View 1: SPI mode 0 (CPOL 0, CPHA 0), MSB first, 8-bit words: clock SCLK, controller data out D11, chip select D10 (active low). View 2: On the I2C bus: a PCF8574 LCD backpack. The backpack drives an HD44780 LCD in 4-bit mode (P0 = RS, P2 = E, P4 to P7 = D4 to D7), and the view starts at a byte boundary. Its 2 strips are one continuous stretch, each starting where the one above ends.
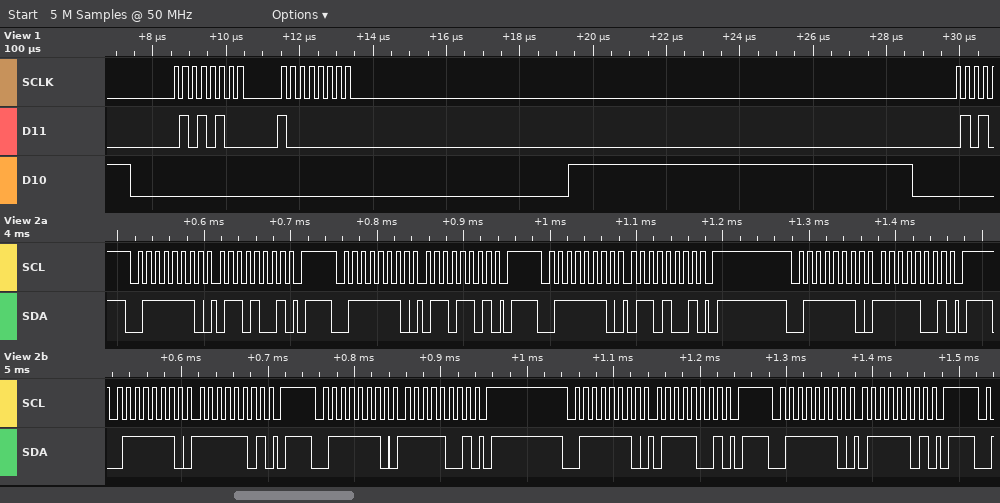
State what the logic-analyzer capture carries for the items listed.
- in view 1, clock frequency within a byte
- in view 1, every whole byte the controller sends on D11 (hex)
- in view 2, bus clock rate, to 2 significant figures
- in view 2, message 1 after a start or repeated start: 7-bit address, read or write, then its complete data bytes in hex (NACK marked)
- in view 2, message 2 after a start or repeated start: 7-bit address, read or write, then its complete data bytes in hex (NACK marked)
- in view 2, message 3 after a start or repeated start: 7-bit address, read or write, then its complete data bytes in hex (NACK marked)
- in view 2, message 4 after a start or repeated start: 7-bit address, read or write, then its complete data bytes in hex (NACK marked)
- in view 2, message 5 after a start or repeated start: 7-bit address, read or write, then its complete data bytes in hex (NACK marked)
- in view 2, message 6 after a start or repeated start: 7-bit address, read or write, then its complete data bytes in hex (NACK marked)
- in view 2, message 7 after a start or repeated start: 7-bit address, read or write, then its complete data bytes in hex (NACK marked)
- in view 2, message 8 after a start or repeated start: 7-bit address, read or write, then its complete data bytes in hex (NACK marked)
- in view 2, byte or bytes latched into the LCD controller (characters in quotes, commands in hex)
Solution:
4 MHz
54 80
100 kHz
0x3F write: 69
0x3F write: 6D
0x3F write: 69
0x3F write: F9
0x3F write: FD
0x3F write: F9
0x3F write: 79
0x3F write: 7D
'o'
